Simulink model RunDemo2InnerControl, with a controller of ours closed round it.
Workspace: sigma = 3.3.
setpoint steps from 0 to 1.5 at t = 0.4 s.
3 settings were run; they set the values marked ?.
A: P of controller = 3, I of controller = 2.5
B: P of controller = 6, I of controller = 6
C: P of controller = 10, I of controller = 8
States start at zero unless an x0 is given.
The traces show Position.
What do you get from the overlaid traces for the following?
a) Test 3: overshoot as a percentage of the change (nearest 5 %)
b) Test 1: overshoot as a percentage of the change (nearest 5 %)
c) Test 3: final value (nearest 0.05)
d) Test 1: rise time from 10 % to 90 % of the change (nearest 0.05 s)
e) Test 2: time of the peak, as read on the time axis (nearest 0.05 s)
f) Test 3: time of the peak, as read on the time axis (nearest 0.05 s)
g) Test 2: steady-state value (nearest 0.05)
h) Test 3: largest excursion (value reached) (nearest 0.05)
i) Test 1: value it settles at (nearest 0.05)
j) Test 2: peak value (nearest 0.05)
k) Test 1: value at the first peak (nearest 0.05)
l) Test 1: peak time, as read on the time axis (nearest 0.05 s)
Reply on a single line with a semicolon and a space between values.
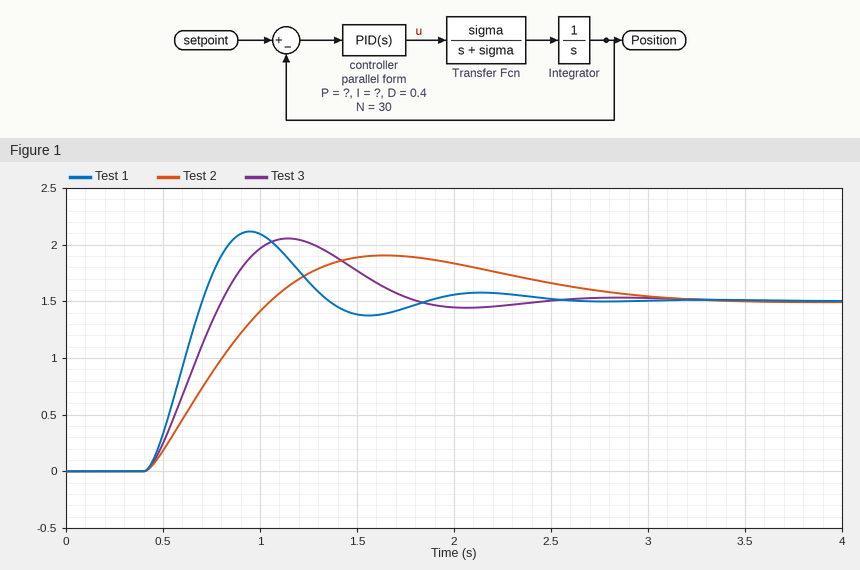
35 %; 40 %; 1.50; 0.20 s; 1.65 s; 1.15 s; 1.50; 2.05; 1.50; 1.90; 2.10; 0.95 s
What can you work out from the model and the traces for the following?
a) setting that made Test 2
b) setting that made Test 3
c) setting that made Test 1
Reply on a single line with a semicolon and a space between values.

A; B; C
